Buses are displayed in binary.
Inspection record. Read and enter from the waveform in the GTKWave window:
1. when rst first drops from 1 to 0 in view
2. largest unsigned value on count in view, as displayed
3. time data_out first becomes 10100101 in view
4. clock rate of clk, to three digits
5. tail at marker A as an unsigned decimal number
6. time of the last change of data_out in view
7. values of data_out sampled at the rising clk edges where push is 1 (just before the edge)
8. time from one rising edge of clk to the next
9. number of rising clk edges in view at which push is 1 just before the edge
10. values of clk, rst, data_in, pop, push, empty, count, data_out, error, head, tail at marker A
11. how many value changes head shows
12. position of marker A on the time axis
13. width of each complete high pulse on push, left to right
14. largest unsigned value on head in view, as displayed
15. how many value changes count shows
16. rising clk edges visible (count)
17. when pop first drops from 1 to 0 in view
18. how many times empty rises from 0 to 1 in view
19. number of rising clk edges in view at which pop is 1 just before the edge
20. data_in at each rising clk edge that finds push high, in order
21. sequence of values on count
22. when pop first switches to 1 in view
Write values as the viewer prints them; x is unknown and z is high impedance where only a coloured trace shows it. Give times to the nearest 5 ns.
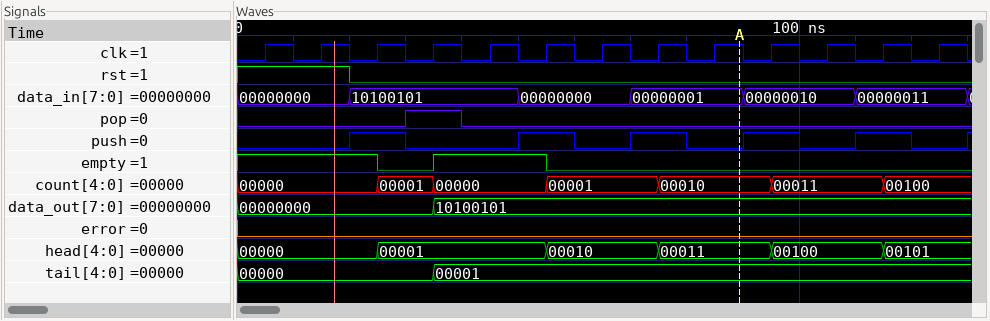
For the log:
20 ns
00100
35 ns
100 MHz
1
35 ns
00000000, 10100101, 10100101, 10100101, 10100101
10 ns
5
clk=1, rst=0, data_in=00000001, pop=0, push=0, empty=0, count=00010, data_out=10100101, error=0, head=00011, tail=00001
5
90 ns
10 ns, 10 ns, 10 ns, 10 ns, 10 ns
00101
6
13
40 ns
1
1
10100101, 00000000, 00000001, 00000010, 00000011
00000, 00001, 00000, 00001, 00010, 00011, 00100
30 ns
